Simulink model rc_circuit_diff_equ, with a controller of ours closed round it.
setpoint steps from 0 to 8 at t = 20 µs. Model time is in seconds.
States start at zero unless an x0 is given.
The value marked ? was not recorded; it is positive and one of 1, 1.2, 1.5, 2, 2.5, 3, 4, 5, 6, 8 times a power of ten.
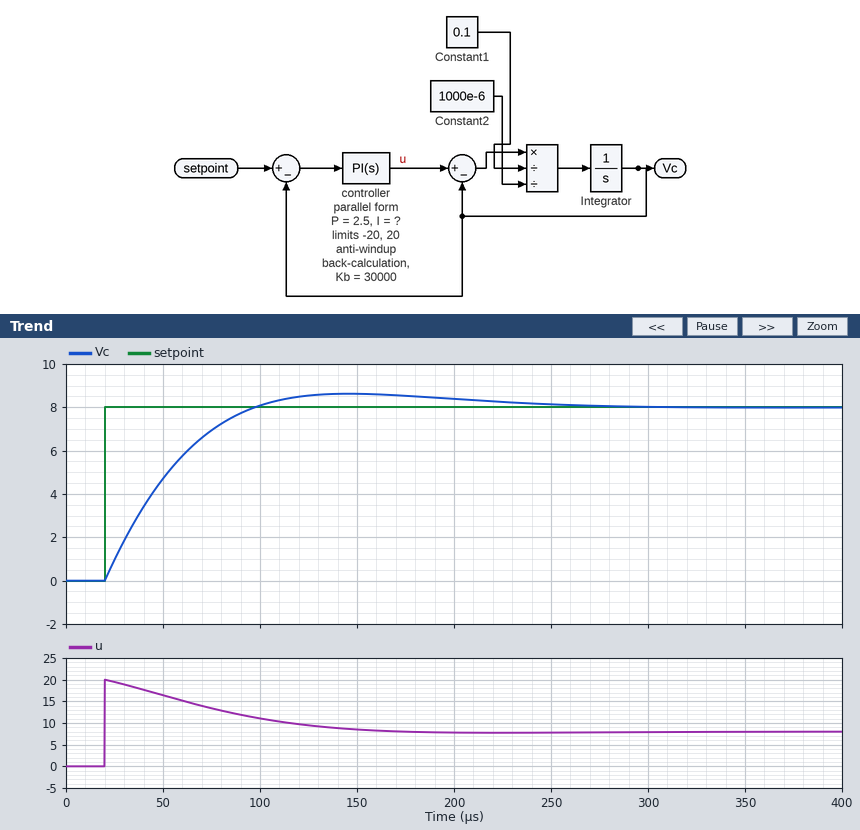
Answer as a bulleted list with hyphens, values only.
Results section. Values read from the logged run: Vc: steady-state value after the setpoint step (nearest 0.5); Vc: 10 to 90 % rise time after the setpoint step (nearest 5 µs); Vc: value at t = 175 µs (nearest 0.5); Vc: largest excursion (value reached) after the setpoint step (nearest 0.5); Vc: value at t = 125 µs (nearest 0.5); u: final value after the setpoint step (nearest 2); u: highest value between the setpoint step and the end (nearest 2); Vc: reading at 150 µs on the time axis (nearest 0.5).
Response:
- 8.0
- 55 µs
- 8.5
- 8.5
- 8.5
- 8
- 20
- 8.5
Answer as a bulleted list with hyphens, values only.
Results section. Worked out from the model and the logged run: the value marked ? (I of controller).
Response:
- 50000
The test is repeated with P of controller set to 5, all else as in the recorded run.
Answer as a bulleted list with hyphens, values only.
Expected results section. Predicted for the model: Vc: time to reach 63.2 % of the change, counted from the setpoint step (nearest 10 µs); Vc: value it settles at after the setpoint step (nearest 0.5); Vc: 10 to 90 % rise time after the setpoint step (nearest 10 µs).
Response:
- 30 µs
- 8.0
- 70 µs
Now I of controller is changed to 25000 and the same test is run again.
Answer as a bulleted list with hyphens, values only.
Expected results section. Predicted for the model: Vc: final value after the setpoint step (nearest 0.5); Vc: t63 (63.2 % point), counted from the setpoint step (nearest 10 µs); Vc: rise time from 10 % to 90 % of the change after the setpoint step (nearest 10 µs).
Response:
- 8.0
- 40 µs
- 90 µs
